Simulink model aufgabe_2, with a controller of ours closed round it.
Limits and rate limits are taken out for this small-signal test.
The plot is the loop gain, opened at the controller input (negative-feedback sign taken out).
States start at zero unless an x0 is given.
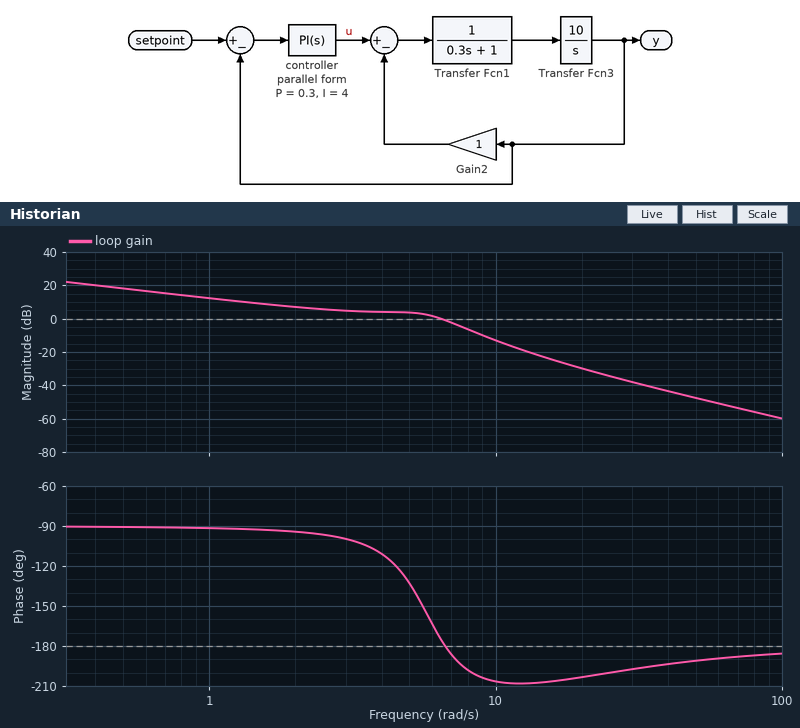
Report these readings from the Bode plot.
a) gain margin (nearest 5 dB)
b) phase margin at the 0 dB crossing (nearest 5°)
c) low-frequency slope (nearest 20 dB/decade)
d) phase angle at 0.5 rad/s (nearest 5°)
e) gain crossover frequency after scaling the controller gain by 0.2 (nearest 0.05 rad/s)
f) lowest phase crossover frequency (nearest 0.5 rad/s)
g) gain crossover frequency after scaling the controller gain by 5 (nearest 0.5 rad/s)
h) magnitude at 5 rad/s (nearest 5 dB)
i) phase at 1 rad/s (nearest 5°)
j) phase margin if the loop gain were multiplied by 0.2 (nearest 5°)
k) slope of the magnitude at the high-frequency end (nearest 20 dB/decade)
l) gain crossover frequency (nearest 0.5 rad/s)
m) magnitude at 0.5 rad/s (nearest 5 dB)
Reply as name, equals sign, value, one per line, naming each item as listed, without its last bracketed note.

gain margin = 0 dB
phase margin at the 0 dB crossing = 5°
low-frequency slope = -20 dB/decade
phase angle at 0.5 rad/s = -90°
gain crossover frequency after scaling the controller gain by 0.2 = 0.80 rad/s
lowest phase crossover frequency = 6.5 rad/s
gain crossover frequency after scaling the controller gain by 5 = 10.5 rad/s
magnitude at 5 rad/s = 5 dB
phase at 1 rad/s = -90°
phase margin if the loop gain were multiplied by 0.2 = 90°
slope of the magnitude at the high-frequency end = -40 dB/decade
gain crossover frequency = 6.5 rad/s
magnitude at 0.5 rad/s = 20 dB
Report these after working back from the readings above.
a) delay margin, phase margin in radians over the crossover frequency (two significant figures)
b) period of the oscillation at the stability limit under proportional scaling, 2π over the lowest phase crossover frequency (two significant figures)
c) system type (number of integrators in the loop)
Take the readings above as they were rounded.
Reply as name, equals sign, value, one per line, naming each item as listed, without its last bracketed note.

delay margin, phase margin in radians over the crossover frequency = 0.013 s
period of the oscillation at the stability limit under proportional scaling, 2π over the lowest phase crossover frequency = 0.97 s
system type = 1
